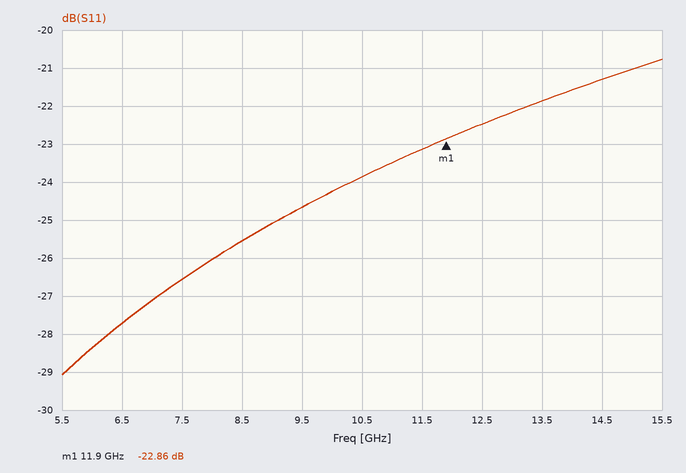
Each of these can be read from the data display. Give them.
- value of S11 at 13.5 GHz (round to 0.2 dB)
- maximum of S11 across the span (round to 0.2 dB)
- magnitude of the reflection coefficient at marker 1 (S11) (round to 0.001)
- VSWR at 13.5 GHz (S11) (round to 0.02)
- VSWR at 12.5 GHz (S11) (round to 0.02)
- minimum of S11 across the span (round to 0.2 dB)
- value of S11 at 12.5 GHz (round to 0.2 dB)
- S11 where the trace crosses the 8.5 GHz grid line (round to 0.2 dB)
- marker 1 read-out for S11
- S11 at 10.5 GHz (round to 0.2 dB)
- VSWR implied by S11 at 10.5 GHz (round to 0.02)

-21.8 dB
-20.8 dB
0.072
1.18
1.16
-29.0 dB
-22.4 dB
-25.6 dB
-22.86 dB
-23.8 dB
1.14
